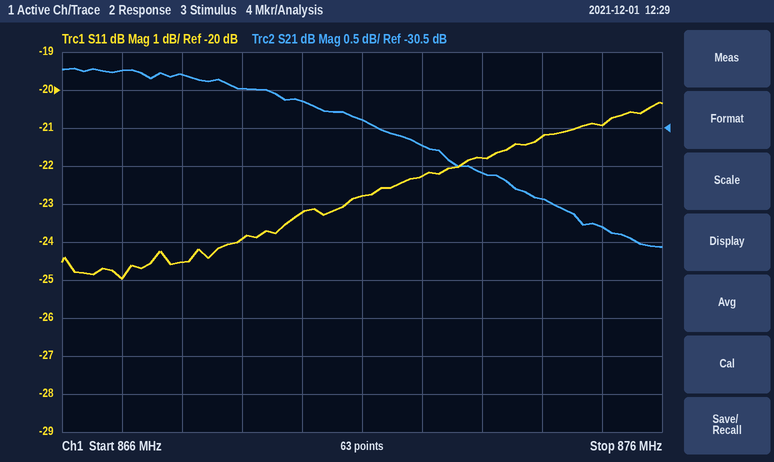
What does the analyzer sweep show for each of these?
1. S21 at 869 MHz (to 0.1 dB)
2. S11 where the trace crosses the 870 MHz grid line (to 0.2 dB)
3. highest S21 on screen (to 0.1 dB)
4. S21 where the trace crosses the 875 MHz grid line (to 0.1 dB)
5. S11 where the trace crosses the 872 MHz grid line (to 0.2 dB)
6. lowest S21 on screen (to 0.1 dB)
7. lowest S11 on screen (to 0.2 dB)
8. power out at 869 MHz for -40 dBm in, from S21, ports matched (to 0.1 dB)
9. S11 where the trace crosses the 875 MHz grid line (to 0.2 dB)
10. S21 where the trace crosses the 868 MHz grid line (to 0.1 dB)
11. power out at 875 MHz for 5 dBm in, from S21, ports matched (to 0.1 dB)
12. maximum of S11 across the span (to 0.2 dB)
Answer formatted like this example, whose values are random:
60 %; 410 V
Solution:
-30.0 dB; -23.2 dB; -29.7 dB; -31.8 dB; -22.2 dB; -32.1 dB; -25.0 dB; -70.0 dBm; -21.0 dB; -29.8 dB; -26.8 dBm; -20.4 dB
